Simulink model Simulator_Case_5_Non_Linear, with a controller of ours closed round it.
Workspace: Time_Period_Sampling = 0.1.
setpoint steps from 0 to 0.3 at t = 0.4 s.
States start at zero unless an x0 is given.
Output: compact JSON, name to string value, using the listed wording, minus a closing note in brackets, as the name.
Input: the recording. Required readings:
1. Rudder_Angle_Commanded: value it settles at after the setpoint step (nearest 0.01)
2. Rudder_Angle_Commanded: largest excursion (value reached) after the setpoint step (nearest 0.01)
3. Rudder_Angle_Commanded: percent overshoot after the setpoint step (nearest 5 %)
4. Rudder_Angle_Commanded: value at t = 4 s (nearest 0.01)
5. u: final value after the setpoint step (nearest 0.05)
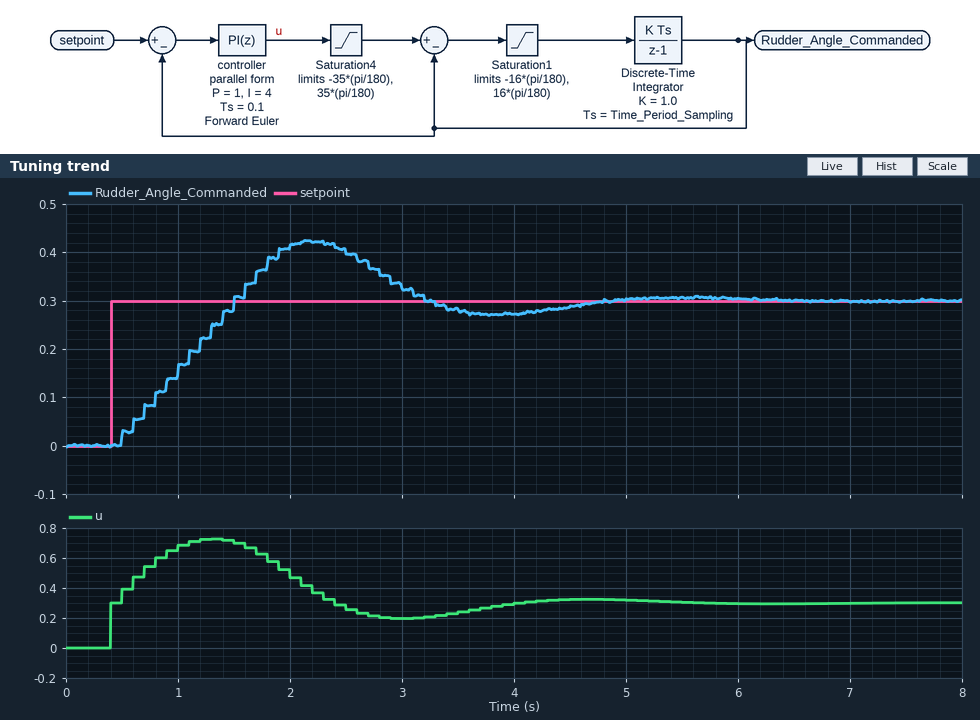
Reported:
{"Rudder_Angle_Commanded: value it settles at after the setpoint step": "0.30", "Rudder_Angle_Commanded: largest excursion (value reached) after the setpoint step": "0.42", "Rudder_Angle_Commanded: percent overshoot after the setpoint step": "40 %", "Rudder_Angle_Commanded: value at t = 4 s": "0.27", "u: final value after the setpoint step": "0.30"}
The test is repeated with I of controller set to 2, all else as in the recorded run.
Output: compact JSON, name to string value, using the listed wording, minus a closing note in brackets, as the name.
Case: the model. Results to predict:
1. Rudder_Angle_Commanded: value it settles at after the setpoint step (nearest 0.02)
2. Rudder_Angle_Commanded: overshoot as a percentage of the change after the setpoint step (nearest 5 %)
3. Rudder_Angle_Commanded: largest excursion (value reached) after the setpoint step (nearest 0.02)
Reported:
{"Rudder_Angle_Commanded: value it settles at after the setpoint step": "0.30", "Rudder_Angle_Commanded: overshoot as a percentage of the change after the setpoint step": "10 %", "Rudder_Angle_Commanded: largest excursion (value reached) after the setpoint step": "0.32"}
